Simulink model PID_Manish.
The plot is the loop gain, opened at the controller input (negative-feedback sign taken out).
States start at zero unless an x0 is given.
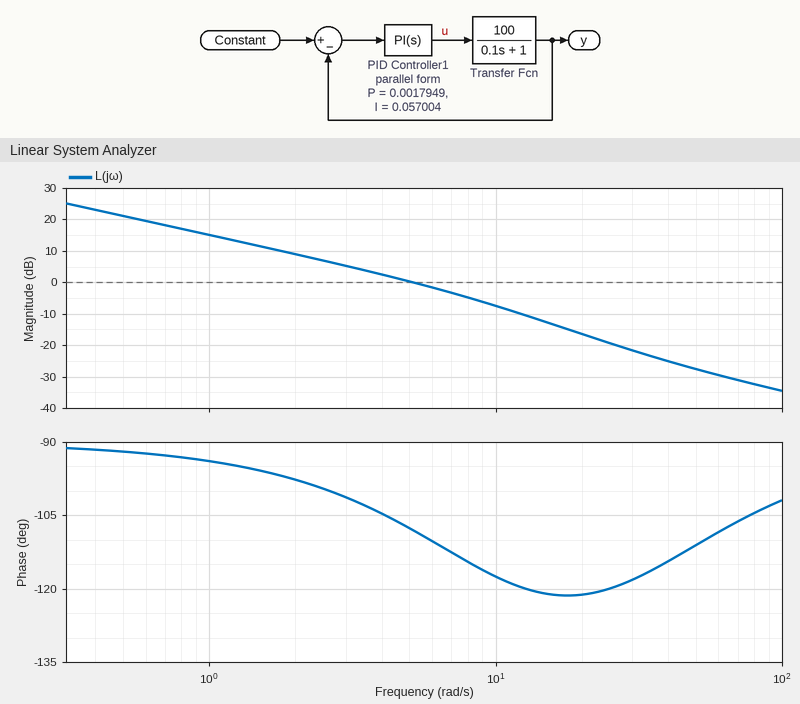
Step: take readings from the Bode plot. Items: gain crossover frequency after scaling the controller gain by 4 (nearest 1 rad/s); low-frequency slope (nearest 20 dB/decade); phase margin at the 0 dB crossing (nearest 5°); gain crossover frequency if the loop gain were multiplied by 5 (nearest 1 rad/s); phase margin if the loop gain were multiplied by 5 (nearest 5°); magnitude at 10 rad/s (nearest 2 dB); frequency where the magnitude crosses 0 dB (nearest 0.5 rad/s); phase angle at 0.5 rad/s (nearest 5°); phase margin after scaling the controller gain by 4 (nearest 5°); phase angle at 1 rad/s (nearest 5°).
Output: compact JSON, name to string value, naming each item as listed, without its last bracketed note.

{"gain crossover frequency after scaling the controller gain by 4": "14 rad/s", "low-frequency slope": "-20 dB/decade", "phase margin at the 0 dB crossing": "70°", "gain crossover frequency if the loop gain were multiplied by 5": "17 rad/s", "phase margin if the loop gain were multiplied by 5": "60°", "magnitude at 10 rad/s": "-8 dB", "frequency where the magnitude crosses 0 dB": "5.0 rad/s", "phase angle at 0.5 rad/s": "-90°", "phase margin after scaling the controller gain by 4": "60°", "phase angle at 1 rad/s": "-95°"}
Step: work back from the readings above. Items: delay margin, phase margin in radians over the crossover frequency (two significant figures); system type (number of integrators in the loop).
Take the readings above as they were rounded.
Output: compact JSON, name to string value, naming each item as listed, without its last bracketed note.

{"delay margin, phase margin in radians over the crossover frequency": "0.24 s", "system type": "1"}
